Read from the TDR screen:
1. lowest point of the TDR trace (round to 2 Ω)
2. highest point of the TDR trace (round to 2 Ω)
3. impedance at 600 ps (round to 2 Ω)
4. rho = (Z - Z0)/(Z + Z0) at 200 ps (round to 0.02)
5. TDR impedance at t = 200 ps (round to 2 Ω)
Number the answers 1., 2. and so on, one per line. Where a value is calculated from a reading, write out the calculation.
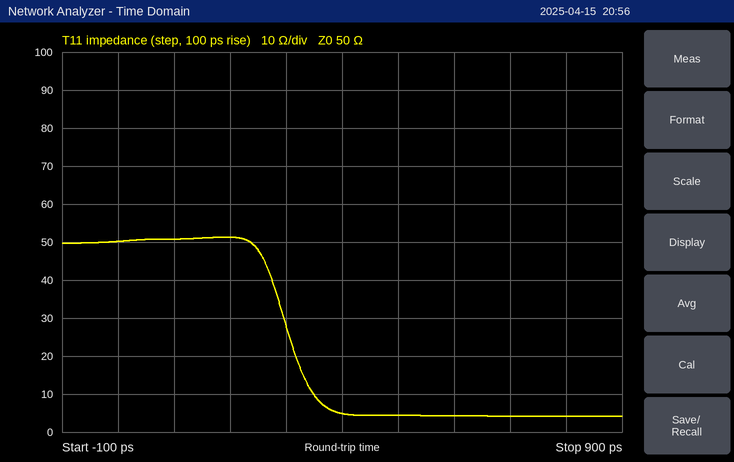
1. 4 Ω
2. 52 Ω
3. 4 Ω
4. (52 − 50)/(52 + 50) ≈ +0.02
5. 52 Ω
